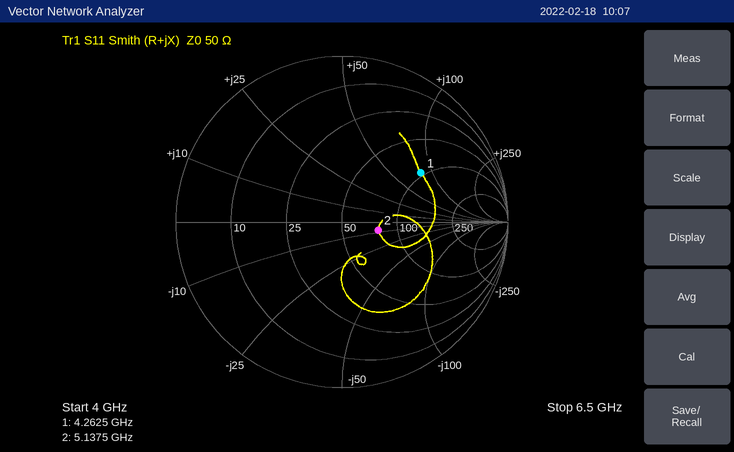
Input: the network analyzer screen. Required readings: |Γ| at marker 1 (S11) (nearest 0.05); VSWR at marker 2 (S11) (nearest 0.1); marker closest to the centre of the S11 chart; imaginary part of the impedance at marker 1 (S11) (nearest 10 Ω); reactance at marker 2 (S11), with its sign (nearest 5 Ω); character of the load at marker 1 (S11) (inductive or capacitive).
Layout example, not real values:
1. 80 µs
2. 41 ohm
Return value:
1. 0.55
2. 1.6
3. marker 2
4. +80 Ω
5. -10 Ω
6. inductive
